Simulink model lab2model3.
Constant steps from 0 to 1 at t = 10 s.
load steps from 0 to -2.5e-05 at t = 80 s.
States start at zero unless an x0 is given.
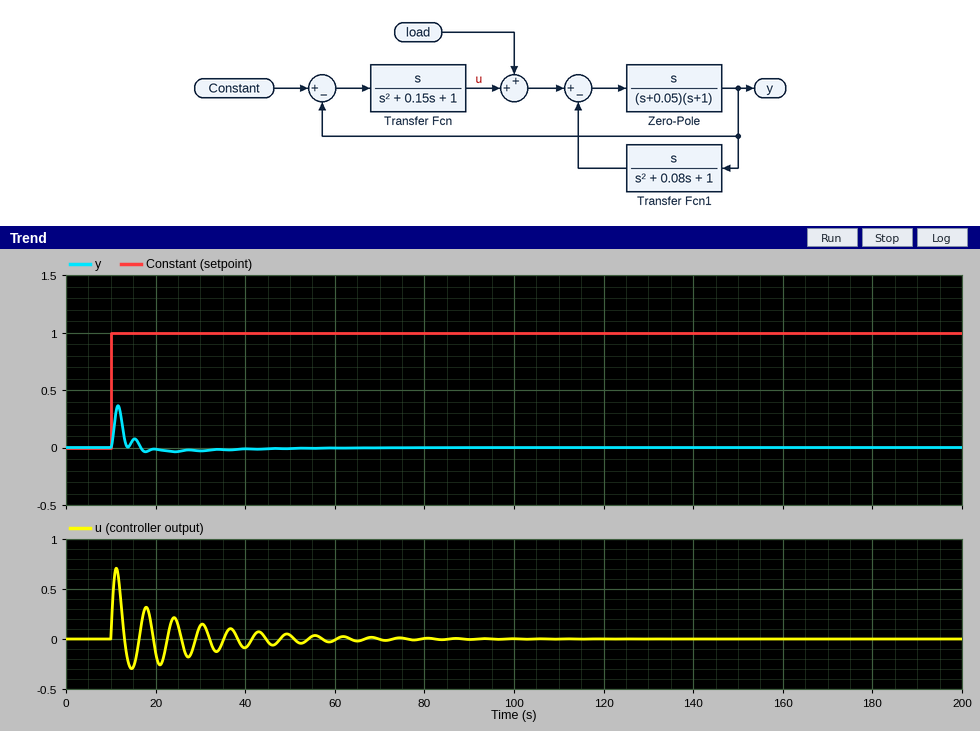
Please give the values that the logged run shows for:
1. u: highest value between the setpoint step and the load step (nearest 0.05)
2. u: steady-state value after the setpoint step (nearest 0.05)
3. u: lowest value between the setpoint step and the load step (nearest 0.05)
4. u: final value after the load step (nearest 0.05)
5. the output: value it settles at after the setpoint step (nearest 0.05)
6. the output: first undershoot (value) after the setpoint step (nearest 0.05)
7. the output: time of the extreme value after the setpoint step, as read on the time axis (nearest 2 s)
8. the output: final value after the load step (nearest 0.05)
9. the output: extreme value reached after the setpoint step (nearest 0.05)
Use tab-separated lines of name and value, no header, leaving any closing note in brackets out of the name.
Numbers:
u: highest value between the setpoint step and the load step	0.70
u: steady-state value after the setpoint step	0.00
u: lowest value between the setpoint step and the load step	-0.30
u: final value after the load step	0.00
the output: value it settles at after the setpoint step	0.00
the output: first undershoot (value) after the setpoint step	0.00
the output: time of the extreme value after the setpoint step, as read on the time axis	12 s
the output: final value after the load step	0.00
the output: extreme value reached after the setpoint step	0.35
